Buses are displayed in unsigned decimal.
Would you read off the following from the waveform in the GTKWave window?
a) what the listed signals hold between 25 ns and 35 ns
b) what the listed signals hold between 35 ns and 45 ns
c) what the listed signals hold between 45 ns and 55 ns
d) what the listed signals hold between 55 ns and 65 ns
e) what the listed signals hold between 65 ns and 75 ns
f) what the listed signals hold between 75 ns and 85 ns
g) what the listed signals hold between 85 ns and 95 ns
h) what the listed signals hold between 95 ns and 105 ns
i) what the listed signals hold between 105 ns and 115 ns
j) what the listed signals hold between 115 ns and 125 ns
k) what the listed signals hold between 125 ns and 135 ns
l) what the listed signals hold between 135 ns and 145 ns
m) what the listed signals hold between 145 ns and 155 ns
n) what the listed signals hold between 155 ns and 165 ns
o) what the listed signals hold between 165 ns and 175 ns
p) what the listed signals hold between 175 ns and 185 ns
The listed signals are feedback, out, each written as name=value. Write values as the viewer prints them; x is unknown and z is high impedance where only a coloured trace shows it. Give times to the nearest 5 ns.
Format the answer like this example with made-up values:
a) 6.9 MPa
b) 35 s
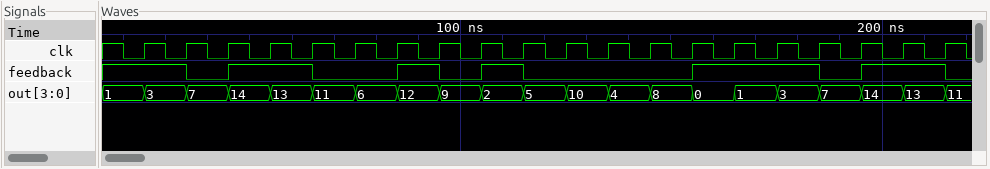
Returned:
a) feedback=1, out=3
b) feedback=0, out=7
c) feedback=1, out=14
d) feedback=1, out=13
e) feedback=0, out=11
f) feedback=0, out=6
g) feedback=1, out=12
h) feedback=0, out=9
i) feedback=1, out=2
j) feedback=0, out=5
k) feedback=0, out=10
l) feedback=0, out=4
m) feedback=0, out=8
n) feedback=1, out=0
o) feedback=1, out=1
p) feedback=1, out=3
